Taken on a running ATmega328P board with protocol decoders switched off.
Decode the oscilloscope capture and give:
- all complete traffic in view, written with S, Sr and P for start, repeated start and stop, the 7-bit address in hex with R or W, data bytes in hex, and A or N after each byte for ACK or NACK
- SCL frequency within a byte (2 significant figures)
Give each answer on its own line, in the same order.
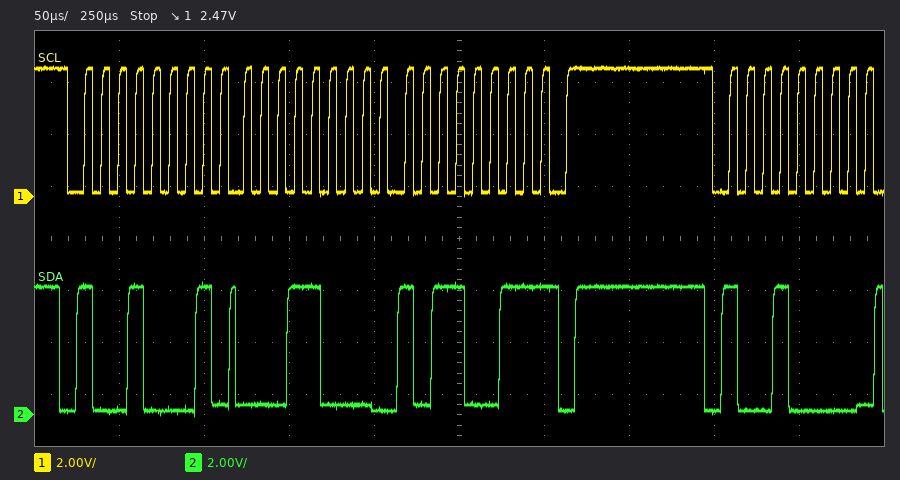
S 48R A 18 A B3 N P S 48W A
100 kHz
